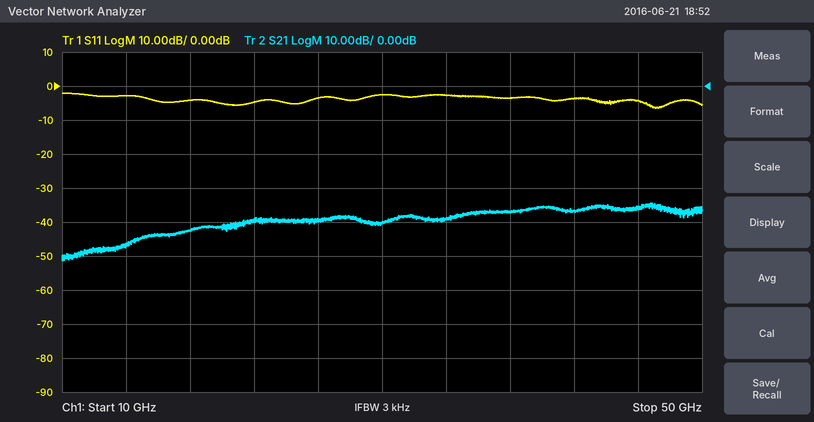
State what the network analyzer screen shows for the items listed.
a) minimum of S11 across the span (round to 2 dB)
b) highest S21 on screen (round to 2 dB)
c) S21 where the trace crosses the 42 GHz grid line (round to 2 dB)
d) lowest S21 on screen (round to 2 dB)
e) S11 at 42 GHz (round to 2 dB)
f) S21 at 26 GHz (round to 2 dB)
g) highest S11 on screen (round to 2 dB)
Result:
-6 dB
-34 dB
-36 dB
-52 dB
-4 dB
-40 dB
-2 dB
